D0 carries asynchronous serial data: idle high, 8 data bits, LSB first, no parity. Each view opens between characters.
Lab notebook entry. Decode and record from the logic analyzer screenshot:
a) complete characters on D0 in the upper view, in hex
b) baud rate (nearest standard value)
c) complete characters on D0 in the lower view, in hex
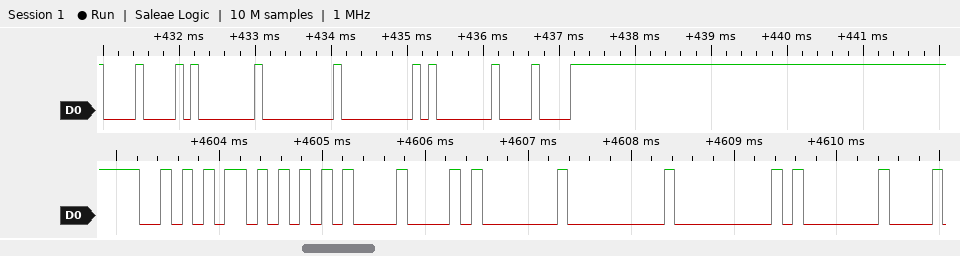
08, 01, 00, 00, 01, 08
9600 baud
AA, 55, 08, 01, 00, 00, 01
